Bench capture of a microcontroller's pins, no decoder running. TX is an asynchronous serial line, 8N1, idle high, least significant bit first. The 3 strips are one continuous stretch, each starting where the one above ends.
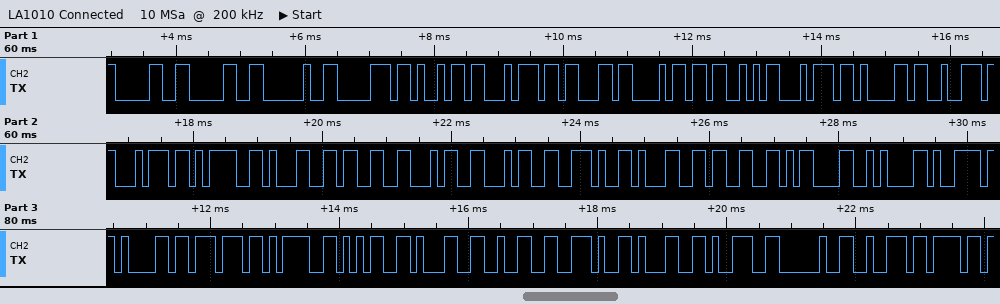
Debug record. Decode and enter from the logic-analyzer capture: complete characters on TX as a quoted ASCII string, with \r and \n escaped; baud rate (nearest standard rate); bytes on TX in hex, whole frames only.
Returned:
"00 pitchStart=1344.13\r\nyaw=512.19 ro"
9600 baud
30 30 20 70 69 74 63 68 53 74 61 72 74 3D 31 33 34 34 2E 31 33 0D 0A 79 61 77 3D 35 31 32 2E 31 39 20 72 6F
